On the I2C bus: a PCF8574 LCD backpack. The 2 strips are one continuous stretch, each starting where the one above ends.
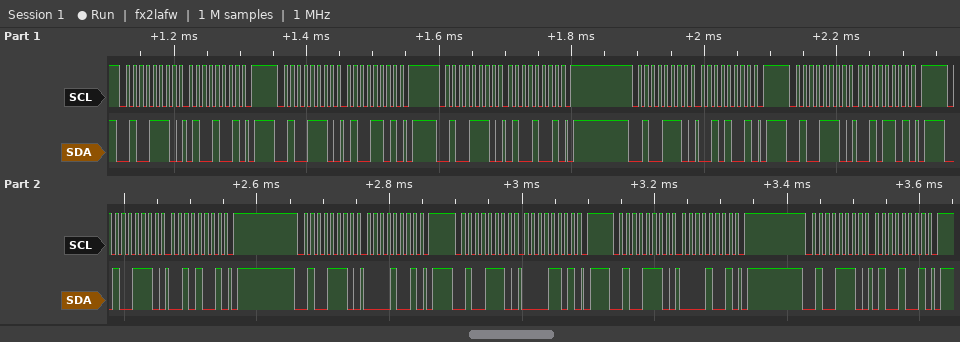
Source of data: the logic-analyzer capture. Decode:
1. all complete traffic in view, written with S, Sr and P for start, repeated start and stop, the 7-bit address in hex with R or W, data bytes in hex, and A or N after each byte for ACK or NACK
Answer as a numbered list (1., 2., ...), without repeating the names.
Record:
1. S 27W A 49 A P S 27W A 4D A P S 27W A 49 A P S 27W A 29 A P S 27W A 2D A P S 27W A 29 A P S 27W A 09 A P S 27W A 0D A P S 27W A 09 A P S 27W A 49 A P
